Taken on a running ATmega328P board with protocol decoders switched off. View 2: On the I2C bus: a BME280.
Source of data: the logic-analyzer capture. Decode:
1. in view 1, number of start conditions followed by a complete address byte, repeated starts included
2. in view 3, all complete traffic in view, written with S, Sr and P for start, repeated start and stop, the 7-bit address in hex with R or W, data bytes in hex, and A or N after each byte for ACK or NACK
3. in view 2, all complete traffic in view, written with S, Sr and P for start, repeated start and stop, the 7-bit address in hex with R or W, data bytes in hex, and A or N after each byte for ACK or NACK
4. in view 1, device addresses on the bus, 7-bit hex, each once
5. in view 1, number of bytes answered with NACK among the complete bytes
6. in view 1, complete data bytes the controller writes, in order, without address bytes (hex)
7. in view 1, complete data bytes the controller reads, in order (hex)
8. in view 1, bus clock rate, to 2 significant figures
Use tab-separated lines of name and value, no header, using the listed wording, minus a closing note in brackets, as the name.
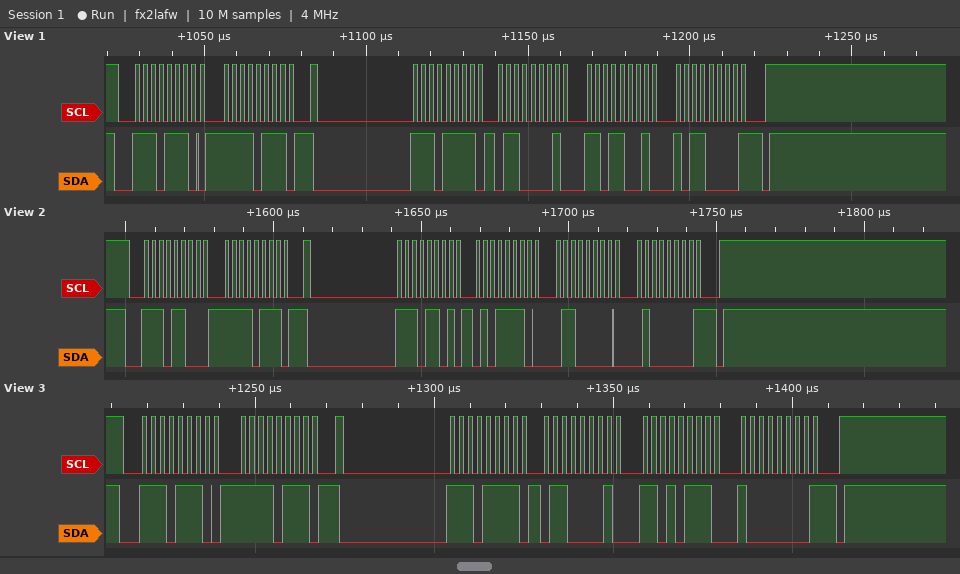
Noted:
in view 1, number of start conditions followed by a complete address byte, repeated starts included	2
in view 3, all complete traffic in view, written with S, Sr and P for start, repeated start and stop, the 7-bit address in hex with R or W, data bytes in hex, and A or N after each byte for ACK or NACK	S 77W A F7 A Sr 77R A 61 A D7 A 80 N P
in view 2, all complete traffic in view, written with S, Sr and P for start, repeated start and stop, the 7-bit address in hex with R or W, data bytes in hex, and A or N after each byte for ACK or NACK	S 76W A F7 A Sr 76R A 5E A 60 A 40 N P
in view 1, device addresses on the bus, 7-bit hex, each once	0x77
in view 1, number of bytes answered with NACK among the complete bytes	1
in view 1, complete data bytes the controller writes, in order, without address bytes	F7
in view 1, complete data bytes the controller reads, in order	61 D9 B0
in view 1, bus clock rate, to 2 significant figures	400 kHz
